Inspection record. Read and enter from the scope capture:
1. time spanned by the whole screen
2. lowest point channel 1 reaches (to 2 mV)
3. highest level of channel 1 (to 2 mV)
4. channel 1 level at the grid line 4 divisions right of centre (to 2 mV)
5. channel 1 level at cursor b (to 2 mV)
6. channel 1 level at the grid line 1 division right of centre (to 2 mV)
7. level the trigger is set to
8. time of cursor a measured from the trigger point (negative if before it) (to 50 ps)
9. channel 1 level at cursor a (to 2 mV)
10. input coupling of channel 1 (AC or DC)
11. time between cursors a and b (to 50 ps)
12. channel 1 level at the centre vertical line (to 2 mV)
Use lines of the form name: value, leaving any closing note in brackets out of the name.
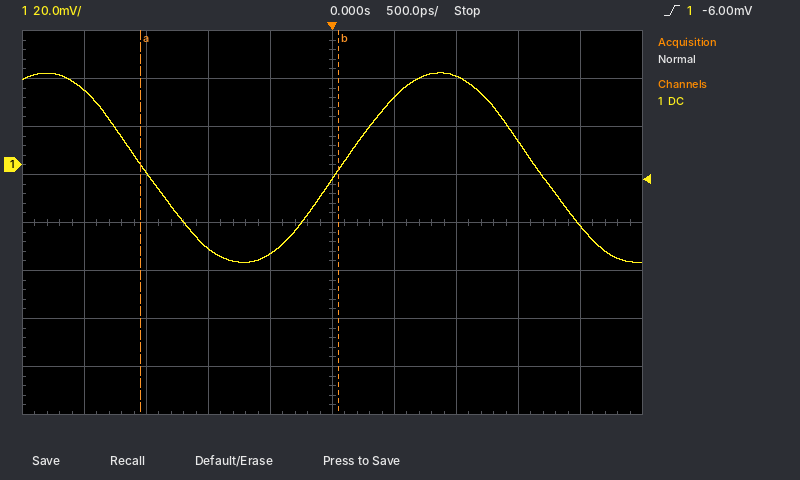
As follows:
time spanned by the whole screen: 5 ns
lowest point channel 1 reaches: -40 mV
highest level of channel 1: 38 mV
channel 1 level at the grid line 4 divisions right of centre: -26 mV
channel 1 level at cursor b: -2 mV
channel 1 level at the grid line 1 division right of centre: 28 mV
level the trigger is set to: -6.00 mV
time of cursor a measured from the trigger point (negative if before it): -1.55 ns
channel 1 level at cursor a: 0 mV
input coupling of channel 1: DC
time between cursors a and b: 1.60 ns
channel 1 level at the centre vertical line: -6 mV
